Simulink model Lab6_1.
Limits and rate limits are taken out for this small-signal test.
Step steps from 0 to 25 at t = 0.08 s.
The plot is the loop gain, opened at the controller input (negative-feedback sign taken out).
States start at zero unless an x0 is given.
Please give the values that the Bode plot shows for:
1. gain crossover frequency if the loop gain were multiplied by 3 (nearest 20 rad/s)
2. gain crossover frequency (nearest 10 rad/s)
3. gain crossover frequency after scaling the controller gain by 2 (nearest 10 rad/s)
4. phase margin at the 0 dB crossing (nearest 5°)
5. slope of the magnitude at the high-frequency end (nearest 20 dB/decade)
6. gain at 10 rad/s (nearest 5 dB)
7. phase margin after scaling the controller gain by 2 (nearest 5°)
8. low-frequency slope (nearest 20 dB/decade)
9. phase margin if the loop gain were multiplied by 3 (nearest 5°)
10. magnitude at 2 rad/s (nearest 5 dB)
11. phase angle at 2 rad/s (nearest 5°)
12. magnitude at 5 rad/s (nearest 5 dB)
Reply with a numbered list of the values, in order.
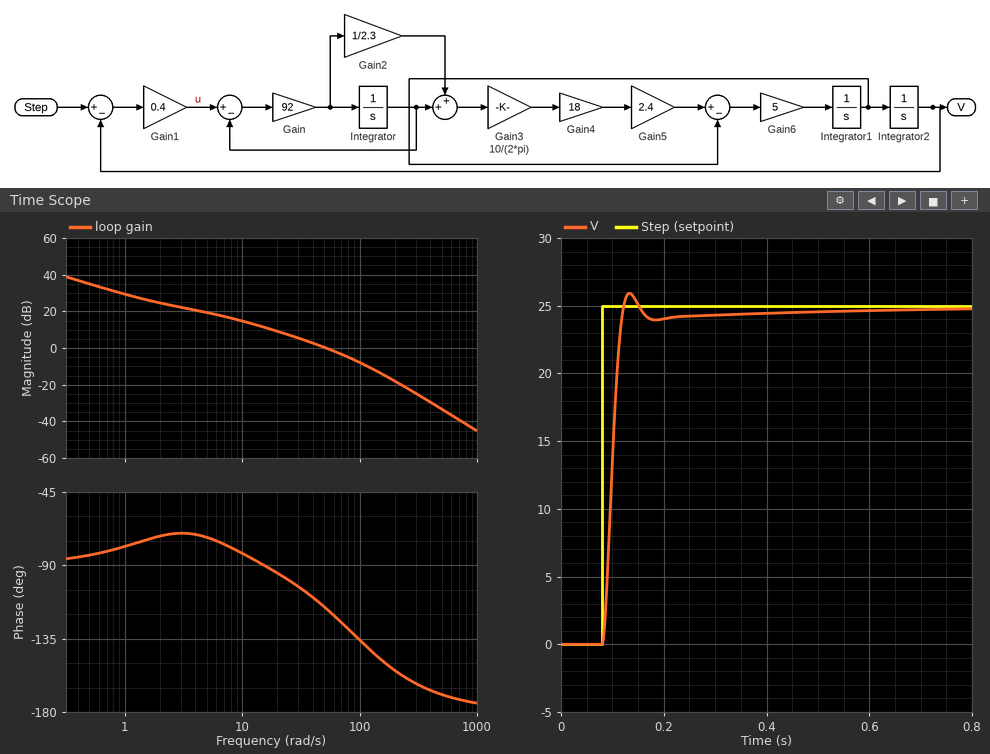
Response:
1. 120 rad/s
2. 50 rad/s
3. 90 rad/s
4. 65°
5. -40 dB/decade
6. 15 dB
7. 50°
8. -20 dB/decade
9. 40°
10. 25 dB
11. -70°
12. 20 dB
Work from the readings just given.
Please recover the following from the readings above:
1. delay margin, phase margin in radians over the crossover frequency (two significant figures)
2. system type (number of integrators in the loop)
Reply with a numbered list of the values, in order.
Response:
1. 0.023 s
2. 1
